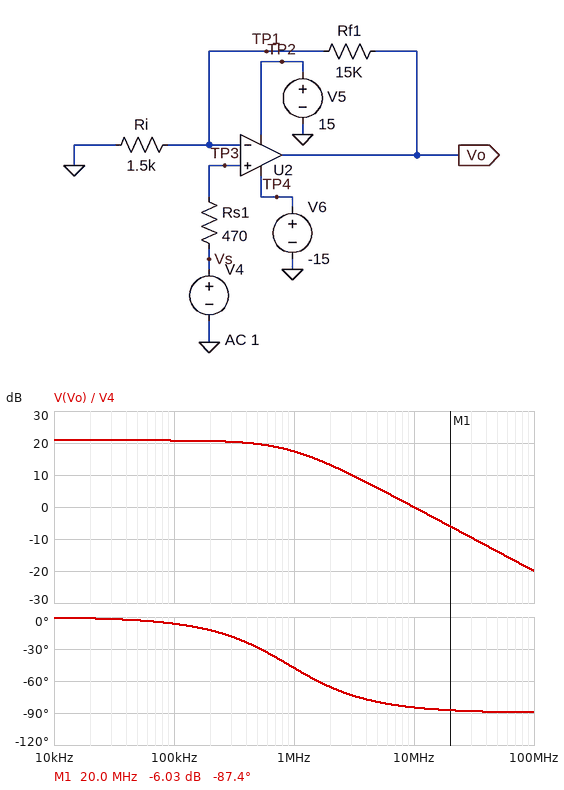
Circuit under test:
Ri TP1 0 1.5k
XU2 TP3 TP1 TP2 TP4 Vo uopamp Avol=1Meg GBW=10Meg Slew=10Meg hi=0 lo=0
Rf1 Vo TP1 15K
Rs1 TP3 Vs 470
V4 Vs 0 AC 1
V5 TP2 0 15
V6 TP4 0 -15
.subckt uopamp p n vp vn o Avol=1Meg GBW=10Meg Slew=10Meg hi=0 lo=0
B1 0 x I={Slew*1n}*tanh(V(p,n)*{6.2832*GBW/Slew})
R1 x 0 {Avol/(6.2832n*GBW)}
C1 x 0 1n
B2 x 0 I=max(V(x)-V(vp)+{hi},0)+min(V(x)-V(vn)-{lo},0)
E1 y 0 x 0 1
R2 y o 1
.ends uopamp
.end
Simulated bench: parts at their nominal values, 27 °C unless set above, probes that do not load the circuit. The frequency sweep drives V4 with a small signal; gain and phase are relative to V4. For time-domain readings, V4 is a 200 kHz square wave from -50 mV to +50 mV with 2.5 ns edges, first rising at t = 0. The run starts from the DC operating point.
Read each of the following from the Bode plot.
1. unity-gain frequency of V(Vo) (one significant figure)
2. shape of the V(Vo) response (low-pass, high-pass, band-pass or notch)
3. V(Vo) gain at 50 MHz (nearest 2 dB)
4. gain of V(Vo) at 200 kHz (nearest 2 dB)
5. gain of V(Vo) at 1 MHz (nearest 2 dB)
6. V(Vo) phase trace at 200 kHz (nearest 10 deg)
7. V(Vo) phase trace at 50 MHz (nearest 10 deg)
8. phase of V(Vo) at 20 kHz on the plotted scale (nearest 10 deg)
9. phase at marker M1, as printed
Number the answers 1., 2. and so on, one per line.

1. 10 MHz
2. low-pass
3. -14 dB
4. 20 dB
5. 18 dB
6. -10 deg
7. -90 deg
8. 0 deg
9. -87.4 deg
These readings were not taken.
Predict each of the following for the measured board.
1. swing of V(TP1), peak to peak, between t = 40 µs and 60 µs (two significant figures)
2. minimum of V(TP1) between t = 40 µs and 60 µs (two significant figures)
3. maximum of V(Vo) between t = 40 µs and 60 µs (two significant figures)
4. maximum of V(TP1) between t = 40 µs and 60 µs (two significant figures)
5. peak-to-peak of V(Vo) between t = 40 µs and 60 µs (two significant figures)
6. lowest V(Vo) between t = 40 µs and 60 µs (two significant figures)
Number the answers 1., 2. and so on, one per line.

1. 100 mV
2. -50 mV
3. 550 mV
4. 50 mV
5. 1.1 V
6. -550 mV
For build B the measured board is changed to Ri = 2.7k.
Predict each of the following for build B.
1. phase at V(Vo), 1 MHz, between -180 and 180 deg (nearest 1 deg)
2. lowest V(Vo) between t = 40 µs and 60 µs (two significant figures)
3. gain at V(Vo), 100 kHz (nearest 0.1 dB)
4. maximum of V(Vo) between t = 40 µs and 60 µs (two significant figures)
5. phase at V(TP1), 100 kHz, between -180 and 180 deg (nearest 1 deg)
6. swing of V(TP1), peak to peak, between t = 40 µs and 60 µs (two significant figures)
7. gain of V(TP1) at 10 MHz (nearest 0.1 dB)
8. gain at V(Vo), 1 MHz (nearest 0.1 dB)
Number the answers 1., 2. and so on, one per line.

1. -33 deg
2. -330 mV
3. 16.3 dB
4. 330 mV
5. -4 deg
6. 100 mV
7. -16.4 dB
8. 14.8 dB
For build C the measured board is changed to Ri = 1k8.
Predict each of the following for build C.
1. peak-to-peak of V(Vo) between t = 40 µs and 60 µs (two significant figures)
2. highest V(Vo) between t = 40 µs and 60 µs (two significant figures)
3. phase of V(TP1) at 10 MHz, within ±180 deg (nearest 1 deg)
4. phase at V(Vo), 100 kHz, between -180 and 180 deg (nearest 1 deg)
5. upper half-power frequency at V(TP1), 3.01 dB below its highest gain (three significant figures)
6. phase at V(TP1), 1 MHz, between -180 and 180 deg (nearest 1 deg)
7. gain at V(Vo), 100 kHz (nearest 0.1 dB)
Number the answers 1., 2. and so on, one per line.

1. 930 mV
2. 470 mV
3. -84 deg
4. -5 deg
5. 1.07 MHz
6. -43 deg
7. 19.4 dB
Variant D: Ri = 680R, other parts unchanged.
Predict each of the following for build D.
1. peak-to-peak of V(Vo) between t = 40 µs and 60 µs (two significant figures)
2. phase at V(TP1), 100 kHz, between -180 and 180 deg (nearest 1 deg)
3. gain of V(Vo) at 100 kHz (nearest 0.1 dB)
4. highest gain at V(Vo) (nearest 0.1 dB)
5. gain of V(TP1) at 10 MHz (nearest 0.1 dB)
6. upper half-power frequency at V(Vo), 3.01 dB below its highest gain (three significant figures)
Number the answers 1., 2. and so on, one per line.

1. 2.3 V
2. -13 deg
3. 27.0 dB
4. 27.3 dB
5. -27.3 dB
6. 434 kHz
